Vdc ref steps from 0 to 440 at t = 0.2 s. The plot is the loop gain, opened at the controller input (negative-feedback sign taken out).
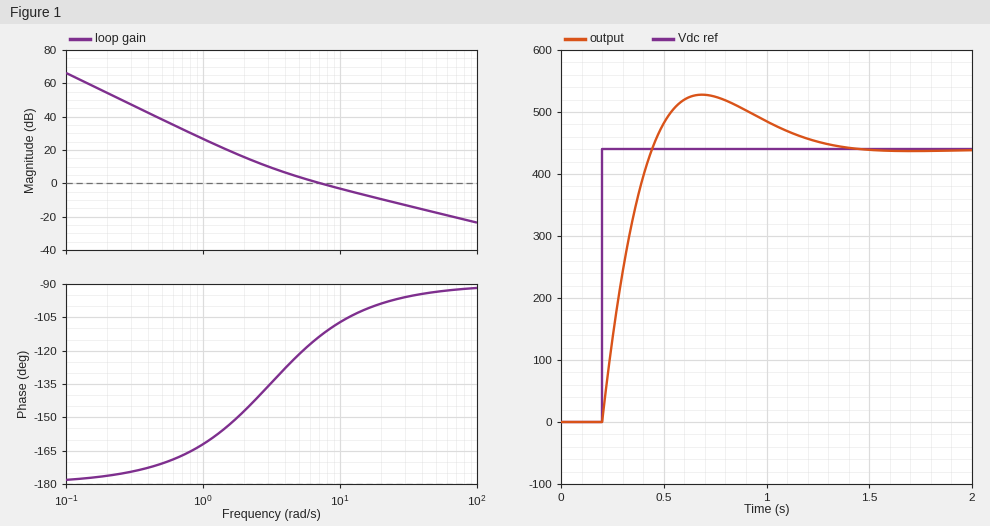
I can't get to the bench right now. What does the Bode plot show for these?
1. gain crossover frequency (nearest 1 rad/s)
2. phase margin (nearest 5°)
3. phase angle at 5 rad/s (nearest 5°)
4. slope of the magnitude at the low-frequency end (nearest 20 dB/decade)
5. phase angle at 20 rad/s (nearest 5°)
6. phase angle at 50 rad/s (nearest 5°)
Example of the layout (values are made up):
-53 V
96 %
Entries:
7 rad/s
65°
-120°
-40 dB/decade
-100°
-95°
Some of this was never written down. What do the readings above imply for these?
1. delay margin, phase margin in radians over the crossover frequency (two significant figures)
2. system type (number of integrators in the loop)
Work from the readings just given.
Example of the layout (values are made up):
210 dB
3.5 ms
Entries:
0.16 s
2
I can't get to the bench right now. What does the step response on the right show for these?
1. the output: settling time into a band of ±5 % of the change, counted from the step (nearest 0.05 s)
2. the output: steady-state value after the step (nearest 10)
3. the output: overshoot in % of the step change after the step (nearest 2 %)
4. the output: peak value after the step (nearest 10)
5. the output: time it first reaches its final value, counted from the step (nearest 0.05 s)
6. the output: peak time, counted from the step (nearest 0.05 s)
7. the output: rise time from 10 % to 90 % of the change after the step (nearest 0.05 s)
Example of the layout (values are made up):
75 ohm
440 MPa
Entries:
0.95 s
440
20 %
530
0.25 s
0.50 s
0.20 s
